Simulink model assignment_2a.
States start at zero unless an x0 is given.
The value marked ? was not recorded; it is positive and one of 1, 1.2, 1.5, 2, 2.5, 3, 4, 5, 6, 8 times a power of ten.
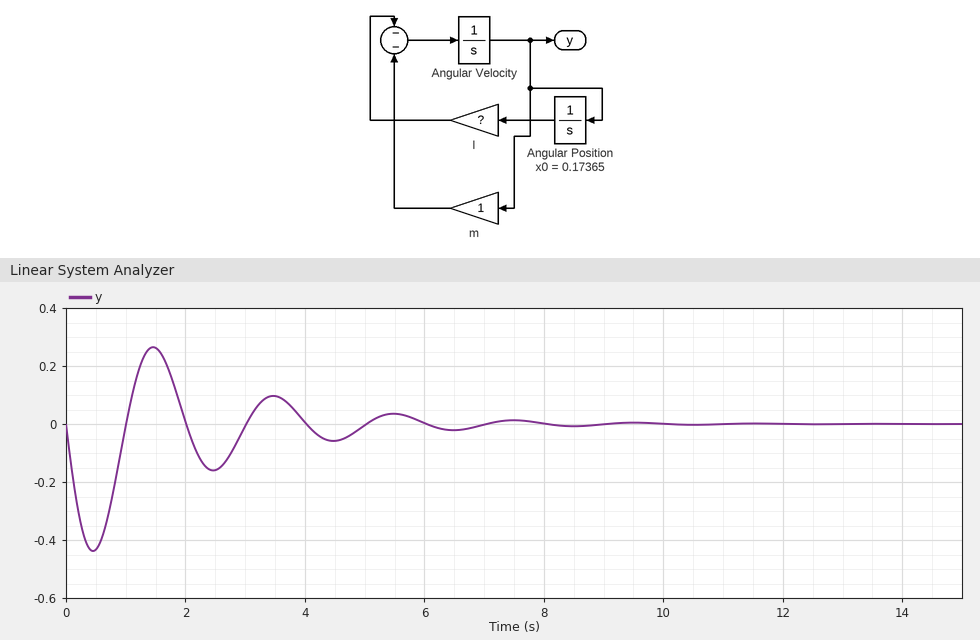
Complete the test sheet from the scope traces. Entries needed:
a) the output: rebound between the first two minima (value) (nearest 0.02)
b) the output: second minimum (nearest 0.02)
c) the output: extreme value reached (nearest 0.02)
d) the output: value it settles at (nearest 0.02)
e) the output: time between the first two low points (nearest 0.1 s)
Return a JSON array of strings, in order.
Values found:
["0.26", "-0.16", "-0.44", "0.00", "2.0 s"]
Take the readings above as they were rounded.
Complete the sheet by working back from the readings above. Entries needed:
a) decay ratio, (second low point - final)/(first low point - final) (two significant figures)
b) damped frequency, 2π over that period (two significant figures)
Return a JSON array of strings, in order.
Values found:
["0.36", "3.1 rad/s"]
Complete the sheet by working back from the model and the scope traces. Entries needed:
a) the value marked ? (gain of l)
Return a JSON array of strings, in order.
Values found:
["10"]
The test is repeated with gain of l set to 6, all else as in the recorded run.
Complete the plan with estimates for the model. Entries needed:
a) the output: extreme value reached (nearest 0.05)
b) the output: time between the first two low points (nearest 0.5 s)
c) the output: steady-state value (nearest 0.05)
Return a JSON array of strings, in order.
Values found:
["-0.30", "2.5 s", "0.00"]
